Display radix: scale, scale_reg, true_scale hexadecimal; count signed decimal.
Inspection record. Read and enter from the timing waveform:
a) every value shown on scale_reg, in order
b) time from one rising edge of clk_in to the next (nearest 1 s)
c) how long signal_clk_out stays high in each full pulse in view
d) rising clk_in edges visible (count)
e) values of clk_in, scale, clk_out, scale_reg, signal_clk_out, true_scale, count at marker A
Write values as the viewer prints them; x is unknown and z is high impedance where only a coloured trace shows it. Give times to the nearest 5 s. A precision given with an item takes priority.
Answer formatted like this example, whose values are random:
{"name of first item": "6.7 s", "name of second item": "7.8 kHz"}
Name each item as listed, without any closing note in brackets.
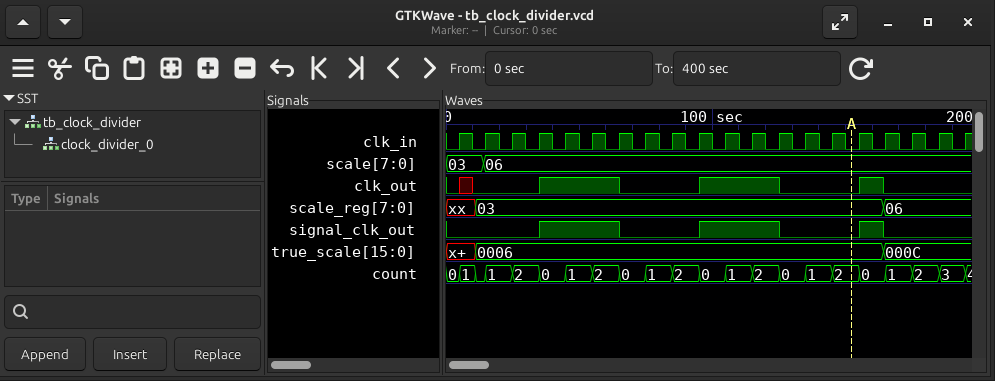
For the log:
{"every value shown on scale_reg, in order": "xx, 03, 06", "time from one rising edge of clk_in to the next": "10 s", "how long signal_clk_out stays high in each full pulse in view": "30 s, 30 s, 10 s", "rising clk_in edges visible": "20", "values of clk_in, scale, clk_out, scale_reg, signal_clk_out, true_scale, count at marker A": "clk_in=0, scale=06, clk_out=0, scale_reg=03, signal_clk_out=0, true_scale=0006, count=2"}
